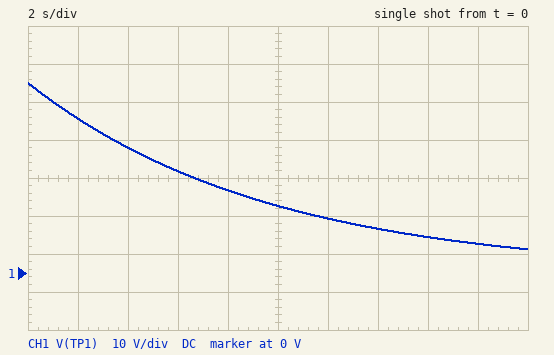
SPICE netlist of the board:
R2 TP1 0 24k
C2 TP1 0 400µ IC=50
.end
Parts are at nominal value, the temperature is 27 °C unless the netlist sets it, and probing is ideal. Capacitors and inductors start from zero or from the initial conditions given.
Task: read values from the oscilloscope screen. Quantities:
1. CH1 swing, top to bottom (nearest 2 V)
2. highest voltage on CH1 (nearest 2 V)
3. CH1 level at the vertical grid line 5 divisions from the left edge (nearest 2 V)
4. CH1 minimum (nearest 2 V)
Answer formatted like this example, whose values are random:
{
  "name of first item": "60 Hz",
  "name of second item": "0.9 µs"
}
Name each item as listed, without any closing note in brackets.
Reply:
{
  "CH1 swing, top to bottom": "44 V",
  "highest voltage on CH1": "50 V",
  "CH1 level at the vertical grid line 5 divisions from the left edge": "18 V",
  "CH1 minimum": "6 V"
}
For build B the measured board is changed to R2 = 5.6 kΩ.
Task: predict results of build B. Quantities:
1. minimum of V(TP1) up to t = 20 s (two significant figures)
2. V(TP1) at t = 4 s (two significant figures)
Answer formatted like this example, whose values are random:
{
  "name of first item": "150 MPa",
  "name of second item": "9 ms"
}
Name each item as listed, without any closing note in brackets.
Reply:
{
  "minimum of V(TP1) up to t = 20 s": "6.6 mV",
  "V(TP1) at t = 4 s": "8.4 V"
}
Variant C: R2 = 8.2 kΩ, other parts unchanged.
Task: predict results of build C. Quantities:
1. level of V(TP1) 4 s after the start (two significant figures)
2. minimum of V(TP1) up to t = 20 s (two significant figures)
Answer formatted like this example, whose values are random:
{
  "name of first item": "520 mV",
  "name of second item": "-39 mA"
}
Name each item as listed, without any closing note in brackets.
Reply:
{
  "level of V(TP1) 4 s after the start": "15 V",
  "minimum of V(TP1) up to t = 20 s": "110 mV"
}
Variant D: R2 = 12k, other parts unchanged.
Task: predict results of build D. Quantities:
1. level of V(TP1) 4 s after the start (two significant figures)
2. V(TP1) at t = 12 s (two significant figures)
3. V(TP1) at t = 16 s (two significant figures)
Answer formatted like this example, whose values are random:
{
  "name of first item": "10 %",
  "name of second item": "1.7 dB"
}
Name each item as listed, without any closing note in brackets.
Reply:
{
  "level of V(TP1) 4 s after the start": "22 V",
  "V(TP1) at t = 12 s": "4.1 V",
  "V(TP1) at t = 16 s": "1.8 V"
}
